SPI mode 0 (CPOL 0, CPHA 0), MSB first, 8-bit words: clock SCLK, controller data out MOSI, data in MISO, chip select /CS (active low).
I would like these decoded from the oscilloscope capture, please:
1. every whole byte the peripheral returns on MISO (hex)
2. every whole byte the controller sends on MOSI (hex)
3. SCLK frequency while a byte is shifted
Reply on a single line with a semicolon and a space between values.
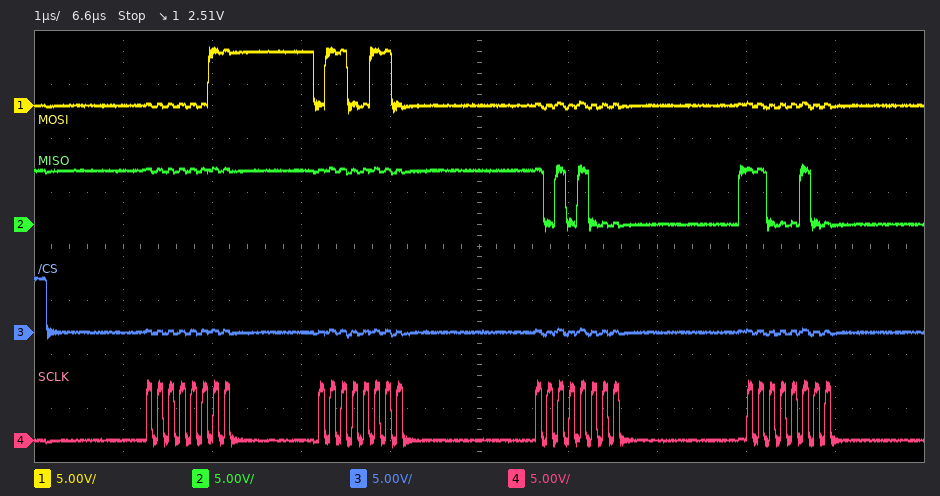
0xFF 0xFF 0xA8 0xC4; 0x03 0x66 0x00 0x00; 8 MHz
